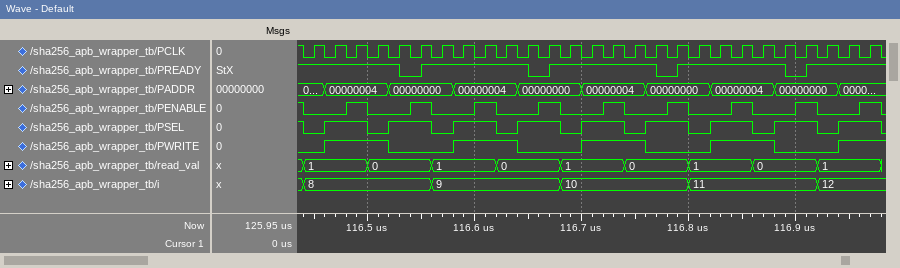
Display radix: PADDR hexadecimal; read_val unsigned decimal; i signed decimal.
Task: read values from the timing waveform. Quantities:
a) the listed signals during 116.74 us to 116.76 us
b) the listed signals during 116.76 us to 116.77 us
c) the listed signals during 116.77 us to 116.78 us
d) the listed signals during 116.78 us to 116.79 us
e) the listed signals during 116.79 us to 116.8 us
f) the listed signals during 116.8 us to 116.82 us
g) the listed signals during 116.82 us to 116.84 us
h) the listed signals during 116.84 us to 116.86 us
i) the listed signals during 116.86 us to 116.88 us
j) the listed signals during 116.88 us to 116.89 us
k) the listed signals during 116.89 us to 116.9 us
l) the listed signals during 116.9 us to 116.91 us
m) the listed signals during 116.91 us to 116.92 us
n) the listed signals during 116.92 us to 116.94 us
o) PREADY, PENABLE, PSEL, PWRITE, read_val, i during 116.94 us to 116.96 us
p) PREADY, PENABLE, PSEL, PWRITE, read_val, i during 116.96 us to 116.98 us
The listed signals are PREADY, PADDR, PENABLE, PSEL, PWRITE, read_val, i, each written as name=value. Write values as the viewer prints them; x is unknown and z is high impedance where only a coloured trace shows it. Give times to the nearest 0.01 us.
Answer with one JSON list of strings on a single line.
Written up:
["PREADY=1, PADDR=00000004, PENABLE=0, PSEL=0, PWRITE=1, read_val=0, i=10", "PREADY=1, PADDR=00000000, PENABLE=0, PSEL=1, PWRITE=0, read_val=0, i=10", "PREADY=0, PADDR=00000000, PENABLE=0, PSEL=1, PWRITE=0, read_val=0, i=10", "PREADY=0, PADDR=00000000, PENABLE=1, PSEL=1, PWRITE=0, read_val=0, i=10", "PREADY=1, PADDR=00000000, PENABLE=1, PSEL=1, PWRITE=0, read_val=0, i=10", "PREADY=1, PADDR=00000000, PENABLE=0, PSEL=0, PWRITE=0, read_val=1, i=11", "PREADY=1, PADDR=00000004, PENABLE=0, PSEL=1, PWRITE=1, read_val=1, i=11", "PREADY=1, PADDR=00000004, PENABLE=1, PSEL=1, PWRITE=1, read_val=1, i=11", "PREADY=1, PADDR=00000004, PENABLE=0, PSEL=0, PWRITE=1, read_val=0, i=11", "PREADY=1, PADDR=00000000, PENABLE=0, PSEL=1, PWRITE=0, read_val=0, i=11", "PREADY=0, PADDR=00000000, PENABLE=0, PSEL=1, PWRITE=0, read_val=0, i=11", "PREADY=0, PADDR=00000000, PENABLE=1, PSEL=1, PWRITE=0, read_val=0, i=11", "PREADY=1, PADDR=00000000, PENABLE=1, PSEL=1, PWRITE=0, read_val=0, i=11", "PREADY=1, PADDR=00000000, PENABLE=0, PSEL=0, PWRITE=0, read_val=1, i=12", "PREADY=1, PENABLE=0, PSEL=1, PWRITE=1, read_val=1, i=12", "PREADY=1, PENABLE=1, PSEL=1, PWRITE=1, read_val=1, i=12"]
